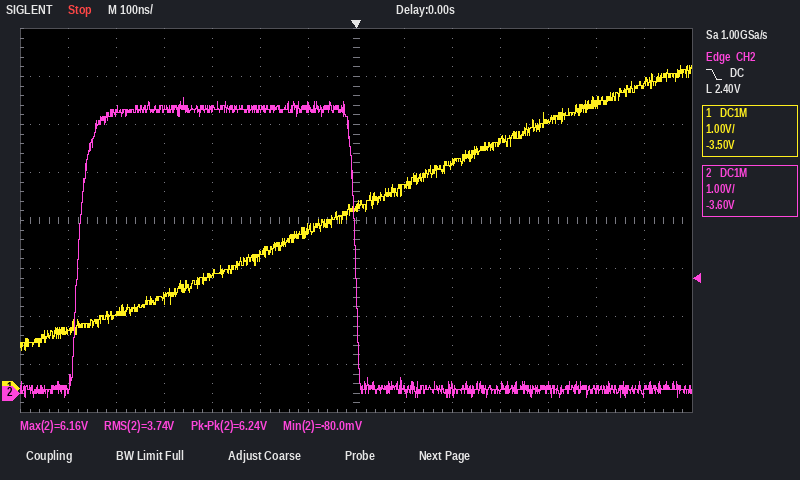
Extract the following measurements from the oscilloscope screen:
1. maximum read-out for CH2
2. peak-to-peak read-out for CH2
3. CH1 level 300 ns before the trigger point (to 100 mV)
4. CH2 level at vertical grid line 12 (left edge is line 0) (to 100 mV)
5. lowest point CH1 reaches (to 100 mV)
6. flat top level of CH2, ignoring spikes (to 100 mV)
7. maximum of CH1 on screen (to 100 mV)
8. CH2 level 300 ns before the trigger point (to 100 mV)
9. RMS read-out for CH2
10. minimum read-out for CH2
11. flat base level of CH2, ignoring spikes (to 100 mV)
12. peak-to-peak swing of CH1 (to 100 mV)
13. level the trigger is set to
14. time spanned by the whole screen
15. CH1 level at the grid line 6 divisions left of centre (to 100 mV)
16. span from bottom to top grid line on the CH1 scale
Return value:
6.16 V
6.24 V
2.4 V
100 mV
800 mV
5.9 V
6.7 V
5.9 V
3.74 V
-80.0 mV
100 mV
5.9 V
2.40 V
1.4 µs
1.2 V
8 V
